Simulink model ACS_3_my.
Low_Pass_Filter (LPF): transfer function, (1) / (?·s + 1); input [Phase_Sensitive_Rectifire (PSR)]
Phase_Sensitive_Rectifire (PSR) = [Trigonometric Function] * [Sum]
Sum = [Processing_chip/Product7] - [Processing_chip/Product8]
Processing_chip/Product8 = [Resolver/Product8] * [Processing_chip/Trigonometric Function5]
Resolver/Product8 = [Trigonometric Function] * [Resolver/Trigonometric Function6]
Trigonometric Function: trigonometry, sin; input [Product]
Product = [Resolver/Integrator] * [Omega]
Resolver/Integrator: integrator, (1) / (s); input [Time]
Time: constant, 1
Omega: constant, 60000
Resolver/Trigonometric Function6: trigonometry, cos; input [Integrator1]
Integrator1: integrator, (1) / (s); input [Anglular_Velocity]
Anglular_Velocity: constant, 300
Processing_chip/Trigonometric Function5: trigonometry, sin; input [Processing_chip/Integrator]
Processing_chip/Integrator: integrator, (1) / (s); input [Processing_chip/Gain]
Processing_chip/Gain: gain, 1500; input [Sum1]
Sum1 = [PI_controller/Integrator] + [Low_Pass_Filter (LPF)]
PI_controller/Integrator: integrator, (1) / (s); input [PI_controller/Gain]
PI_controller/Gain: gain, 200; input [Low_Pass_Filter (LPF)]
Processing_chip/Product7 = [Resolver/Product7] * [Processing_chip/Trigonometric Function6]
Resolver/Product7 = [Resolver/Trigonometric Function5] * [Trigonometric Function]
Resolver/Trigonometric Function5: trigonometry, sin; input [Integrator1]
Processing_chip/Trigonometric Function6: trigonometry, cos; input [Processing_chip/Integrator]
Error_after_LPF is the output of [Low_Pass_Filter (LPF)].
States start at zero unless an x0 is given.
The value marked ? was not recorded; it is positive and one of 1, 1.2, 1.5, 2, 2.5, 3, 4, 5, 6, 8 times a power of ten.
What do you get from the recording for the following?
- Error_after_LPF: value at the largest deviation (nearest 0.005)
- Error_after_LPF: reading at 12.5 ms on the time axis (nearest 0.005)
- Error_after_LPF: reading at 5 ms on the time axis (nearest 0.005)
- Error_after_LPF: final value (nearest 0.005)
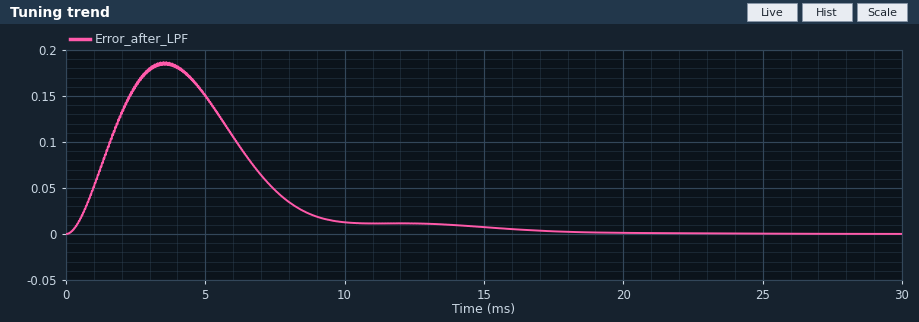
0.185
0.010
0.150
0.000
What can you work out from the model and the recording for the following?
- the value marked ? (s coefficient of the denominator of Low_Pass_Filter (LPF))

0.001
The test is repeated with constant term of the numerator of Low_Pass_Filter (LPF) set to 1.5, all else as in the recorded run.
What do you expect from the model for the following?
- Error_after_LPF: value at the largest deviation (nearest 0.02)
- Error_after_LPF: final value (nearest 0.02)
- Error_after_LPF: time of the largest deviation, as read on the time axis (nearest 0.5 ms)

0.20
0.00
3.0 ms
